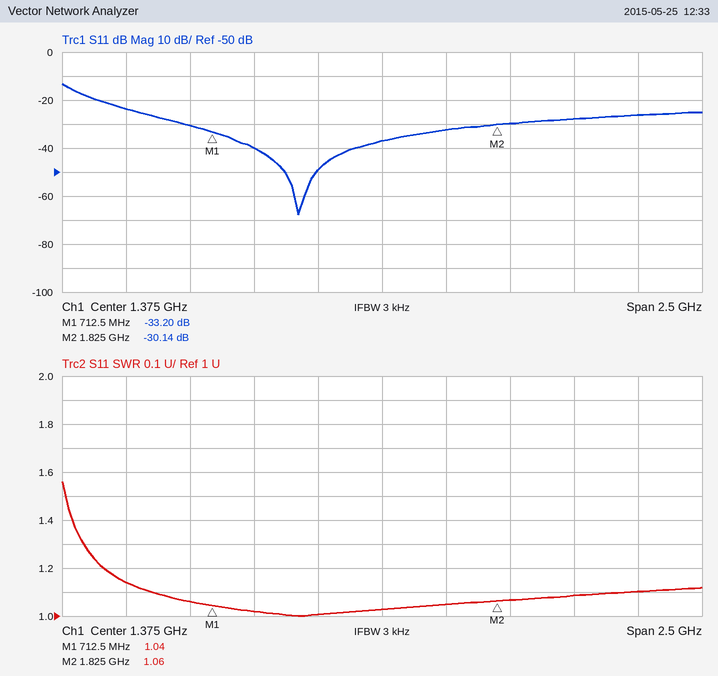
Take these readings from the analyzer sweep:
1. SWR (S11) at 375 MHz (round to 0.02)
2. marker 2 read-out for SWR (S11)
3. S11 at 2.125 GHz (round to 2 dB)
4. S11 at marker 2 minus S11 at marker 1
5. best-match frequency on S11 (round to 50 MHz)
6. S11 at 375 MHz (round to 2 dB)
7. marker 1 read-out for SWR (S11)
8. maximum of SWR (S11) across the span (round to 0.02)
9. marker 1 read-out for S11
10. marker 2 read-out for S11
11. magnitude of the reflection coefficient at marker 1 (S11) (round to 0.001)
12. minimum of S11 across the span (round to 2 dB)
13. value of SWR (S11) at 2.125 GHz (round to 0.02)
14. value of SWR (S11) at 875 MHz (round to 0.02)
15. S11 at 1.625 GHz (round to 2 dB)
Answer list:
1.14
1.06
-28 dB
3.06 dB
1.05 GHz
-24 dB
1.04
1.56
-33.20 dB
-30.14 dB
0.022
-68 dB
1.08
1.02
-32 dB
